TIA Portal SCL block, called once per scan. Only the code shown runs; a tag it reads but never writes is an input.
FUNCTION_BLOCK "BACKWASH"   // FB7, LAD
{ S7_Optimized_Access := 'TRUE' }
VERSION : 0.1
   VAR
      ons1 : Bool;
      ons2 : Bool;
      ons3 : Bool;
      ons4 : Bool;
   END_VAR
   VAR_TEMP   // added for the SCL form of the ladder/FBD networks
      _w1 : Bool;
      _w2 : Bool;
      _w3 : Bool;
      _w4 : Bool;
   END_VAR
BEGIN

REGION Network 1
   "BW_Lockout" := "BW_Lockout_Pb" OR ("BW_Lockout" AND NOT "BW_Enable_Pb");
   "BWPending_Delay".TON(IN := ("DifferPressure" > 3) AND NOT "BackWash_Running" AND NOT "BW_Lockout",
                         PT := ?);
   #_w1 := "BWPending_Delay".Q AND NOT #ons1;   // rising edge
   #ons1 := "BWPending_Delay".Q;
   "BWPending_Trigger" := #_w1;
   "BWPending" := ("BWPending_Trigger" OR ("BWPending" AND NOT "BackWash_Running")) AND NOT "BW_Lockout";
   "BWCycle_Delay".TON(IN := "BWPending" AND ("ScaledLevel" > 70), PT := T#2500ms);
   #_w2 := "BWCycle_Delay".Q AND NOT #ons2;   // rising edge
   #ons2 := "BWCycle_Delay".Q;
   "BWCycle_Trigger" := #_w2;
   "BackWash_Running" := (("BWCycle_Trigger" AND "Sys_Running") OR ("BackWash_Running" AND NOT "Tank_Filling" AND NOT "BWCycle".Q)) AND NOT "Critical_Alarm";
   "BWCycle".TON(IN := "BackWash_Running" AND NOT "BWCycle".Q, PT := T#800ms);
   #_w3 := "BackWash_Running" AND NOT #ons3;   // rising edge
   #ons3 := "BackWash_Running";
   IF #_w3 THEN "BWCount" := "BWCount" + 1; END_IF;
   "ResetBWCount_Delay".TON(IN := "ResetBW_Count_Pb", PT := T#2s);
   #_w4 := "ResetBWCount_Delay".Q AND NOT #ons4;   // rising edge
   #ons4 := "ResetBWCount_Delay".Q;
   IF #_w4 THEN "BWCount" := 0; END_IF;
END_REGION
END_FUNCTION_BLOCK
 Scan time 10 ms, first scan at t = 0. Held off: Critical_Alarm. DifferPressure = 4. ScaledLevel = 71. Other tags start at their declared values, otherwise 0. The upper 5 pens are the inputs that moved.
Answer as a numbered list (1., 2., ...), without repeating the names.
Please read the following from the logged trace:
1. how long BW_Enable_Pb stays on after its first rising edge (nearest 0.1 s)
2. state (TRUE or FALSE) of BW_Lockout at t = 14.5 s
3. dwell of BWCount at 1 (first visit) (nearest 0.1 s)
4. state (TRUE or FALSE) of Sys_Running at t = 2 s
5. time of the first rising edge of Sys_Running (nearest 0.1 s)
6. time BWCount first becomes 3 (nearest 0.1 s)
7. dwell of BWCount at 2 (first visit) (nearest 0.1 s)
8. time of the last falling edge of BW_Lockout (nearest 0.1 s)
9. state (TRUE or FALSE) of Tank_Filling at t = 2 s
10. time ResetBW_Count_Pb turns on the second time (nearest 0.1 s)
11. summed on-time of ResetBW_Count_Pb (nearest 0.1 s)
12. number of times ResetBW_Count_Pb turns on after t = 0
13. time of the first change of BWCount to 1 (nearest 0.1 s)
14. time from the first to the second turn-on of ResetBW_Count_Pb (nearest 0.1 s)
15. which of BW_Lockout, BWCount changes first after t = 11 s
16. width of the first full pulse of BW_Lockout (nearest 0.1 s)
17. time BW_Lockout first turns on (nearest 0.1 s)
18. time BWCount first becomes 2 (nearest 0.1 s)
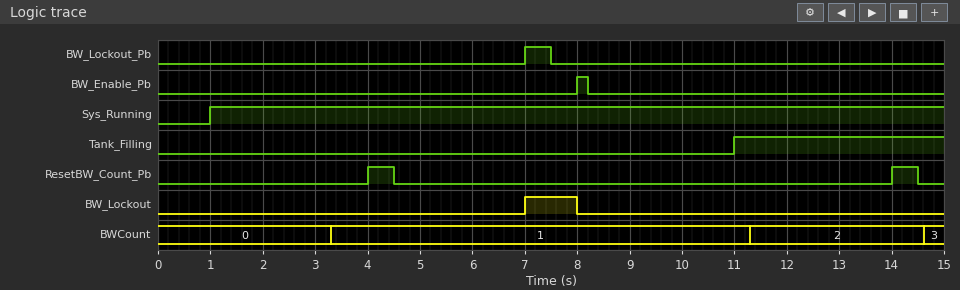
1. 0.2 s
2. FALSE
3. 8.0 s
4. TRUE
5. 1.0 s
6. 14.6 s
7. 3.3 s
8. 8.0 s
9. FALSE
10. 14.0 s
11. 1.0 s
12. 2
13. 3.3 s
14. 10.0 s
15. BWCount
16. 1.0 s
17. 7.0 s
18. 11.3 s
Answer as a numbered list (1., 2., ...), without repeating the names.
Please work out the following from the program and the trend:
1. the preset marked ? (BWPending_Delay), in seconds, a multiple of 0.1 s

1. 0.8 s
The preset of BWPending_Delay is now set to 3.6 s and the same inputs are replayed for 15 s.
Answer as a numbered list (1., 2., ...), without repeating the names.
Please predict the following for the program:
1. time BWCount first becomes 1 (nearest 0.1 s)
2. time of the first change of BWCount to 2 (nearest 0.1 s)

1. 6.1 s
2. 14.1 s
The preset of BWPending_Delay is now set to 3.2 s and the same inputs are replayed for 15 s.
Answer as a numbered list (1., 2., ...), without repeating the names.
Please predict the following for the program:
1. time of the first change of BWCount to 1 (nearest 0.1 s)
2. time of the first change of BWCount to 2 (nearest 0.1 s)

1. 5.7 s
2. 13.7 s
